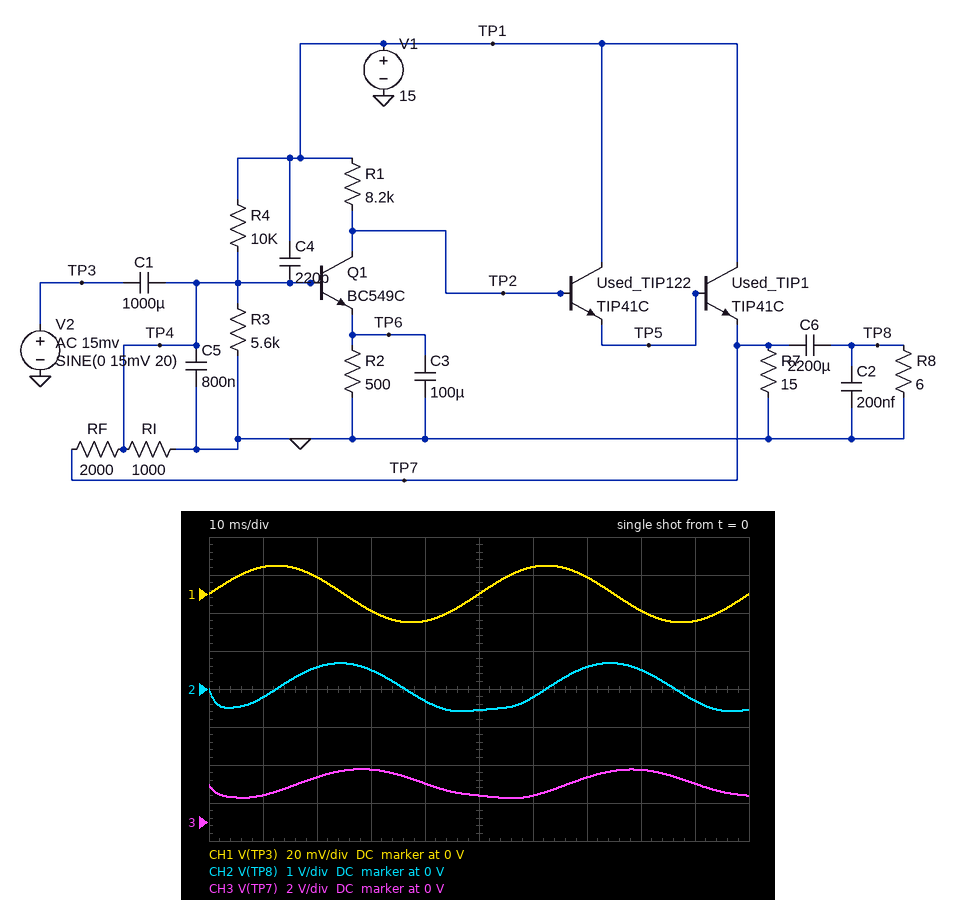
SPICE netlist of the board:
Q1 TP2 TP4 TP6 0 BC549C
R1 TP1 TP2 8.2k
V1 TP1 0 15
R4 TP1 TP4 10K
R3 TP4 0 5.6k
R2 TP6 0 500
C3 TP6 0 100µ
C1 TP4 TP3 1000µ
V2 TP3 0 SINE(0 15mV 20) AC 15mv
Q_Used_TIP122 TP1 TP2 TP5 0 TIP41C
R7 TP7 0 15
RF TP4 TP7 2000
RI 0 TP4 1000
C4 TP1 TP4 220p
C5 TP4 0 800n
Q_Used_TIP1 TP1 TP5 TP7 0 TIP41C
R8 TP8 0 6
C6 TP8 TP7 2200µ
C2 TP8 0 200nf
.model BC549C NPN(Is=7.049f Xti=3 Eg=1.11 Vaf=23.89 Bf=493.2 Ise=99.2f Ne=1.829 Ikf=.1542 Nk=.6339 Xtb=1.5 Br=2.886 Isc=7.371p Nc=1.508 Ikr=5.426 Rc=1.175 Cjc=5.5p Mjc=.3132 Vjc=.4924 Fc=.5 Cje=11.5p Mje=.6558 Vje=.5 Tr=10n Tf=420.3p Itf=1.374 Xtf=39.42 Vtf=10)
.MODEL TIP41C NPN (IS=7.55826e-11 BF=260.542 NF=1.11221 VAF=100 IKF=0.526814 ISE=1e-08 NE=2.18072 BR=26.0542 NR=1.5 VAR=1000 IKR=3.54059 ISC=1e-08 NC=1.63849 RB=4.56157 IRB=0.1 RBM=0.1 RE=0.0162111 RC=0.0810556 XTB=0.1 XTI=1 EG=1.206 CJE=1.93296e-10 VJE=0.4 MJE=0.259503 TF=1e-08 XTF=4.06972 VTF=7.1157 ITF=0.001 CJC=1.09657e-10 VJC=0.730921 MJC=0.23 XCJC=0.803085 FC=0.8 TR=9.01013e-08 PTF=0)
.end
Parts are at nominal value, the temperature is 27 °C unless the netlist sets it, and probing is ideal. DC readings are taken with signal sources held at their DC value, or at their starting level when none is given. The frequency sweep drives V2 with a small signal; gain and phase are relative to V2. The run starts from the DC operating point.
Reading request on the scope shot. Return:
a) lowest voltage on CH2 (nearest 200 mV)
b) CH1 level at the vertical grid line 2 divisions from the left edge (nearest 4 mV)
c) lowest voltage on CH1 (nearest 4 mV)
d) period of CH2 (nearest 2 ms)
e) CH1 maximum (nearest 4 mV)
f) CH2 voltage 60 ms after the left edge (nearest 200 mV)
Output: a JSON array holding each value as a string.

["-600 mV", "8 mV", "-16 mV", "50 ms", "16 mV", "-200 mV"]
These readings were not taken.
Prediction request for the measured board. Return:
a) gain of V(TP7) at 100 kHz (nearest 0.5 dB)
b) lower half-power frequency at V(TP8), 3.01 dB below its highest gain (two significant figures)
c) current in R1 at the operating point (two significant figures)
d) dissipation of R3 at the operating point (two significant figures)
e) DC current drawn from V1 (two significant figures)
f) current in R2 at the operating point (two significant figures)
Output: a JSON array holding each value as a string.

["48.5 dB", "130 Hz", "1.5 mA", "340 µW", "130 mA", "1.4 mA"]
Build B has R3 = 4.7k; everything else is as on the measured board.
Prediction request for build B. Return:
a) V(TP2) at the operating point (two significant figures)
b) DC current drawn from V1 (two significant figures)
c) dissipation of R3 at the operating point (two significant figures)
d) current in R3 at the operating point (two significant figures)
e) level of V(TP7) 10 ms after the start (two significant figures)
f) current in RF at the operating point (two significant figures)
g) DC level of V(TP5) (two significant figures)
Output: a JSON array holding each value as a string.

["3.1 V", "140 mA", "400 µW", "290 µA", "1.5 V", "310 µA", "2.6 V"]
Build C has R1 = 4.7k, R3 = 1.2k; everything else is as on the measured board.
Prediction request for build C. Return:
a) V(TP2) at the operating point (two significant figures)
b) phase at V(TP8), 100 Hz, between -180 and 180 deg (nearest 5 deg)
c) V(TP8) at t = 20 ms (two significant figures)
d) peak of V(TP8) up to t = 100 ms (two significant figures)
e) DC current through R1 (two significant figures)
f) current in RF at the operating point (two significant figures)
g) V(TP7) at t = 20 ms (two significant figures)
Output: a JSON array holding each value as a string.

["6.0 V", "-130 deg", "430 mV", "510 mV", "1.9 mA", "1.6 mA", "5.1 V"]
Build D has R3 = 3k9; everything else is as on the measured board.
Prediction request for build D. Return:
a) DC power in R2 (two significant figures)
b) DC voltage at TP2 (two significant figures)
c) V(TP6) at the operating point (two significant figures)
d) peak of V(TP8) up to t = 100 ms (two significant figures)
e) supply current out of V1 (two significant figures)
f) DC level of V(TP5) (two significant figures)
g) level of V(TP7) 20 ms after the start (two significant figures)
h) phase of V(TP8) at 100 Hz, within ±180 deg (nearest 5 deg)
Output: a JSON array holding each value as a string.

["980 µW", "3.2 V", "700 mV", "690 mV", "140 mA", "2.7 V", "2.5 V", "-135 deg"]
